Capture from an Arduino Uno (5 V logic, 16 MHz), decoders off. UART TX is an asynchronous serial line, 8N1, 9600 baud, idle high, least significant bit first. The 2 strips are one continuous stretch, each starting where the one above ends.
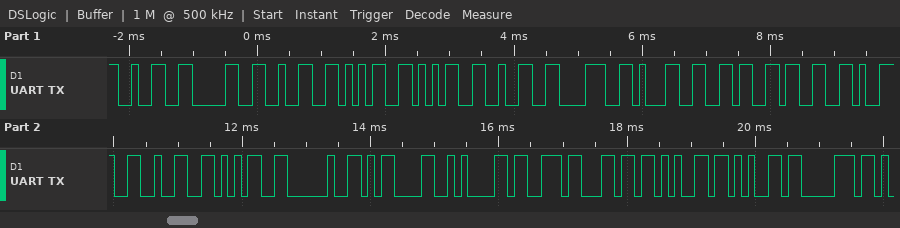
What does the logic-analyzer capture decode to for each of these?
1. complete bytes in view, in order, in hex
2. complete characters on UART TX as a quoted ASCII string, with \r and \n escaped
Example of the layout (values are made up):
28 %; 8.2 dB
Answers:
32 30 32 35 35 32 38 31 36 33 39 32 35 20 0D 0A 73 6C 65 65 70; "2025528163925 \r\nsleep"
